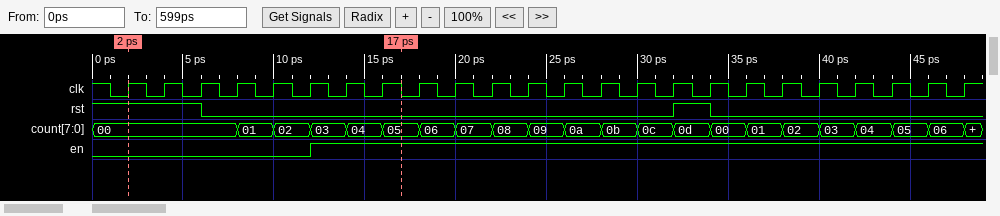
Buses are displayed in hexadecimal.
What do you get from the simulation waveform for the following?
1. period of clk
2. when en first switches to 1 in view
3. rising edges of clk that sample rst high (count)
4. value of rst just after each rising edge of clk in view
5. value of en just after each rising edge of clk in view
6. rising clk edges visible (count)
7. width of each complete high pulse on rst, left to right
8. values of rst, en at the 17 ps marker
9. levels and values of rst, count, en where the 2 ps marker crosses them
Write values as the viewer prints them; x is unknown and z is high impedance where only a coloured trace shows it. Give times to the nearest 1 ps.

2 ps
12 ps
4
1 1 0 0 0 0 0 0 0 0 0 0 0 0 0 1 0 0 0 0 0 0 0 0
0 0 0 0 0 1 1 1 1 1 1 1 1 1 1 1 1 1 1 1 1 1 1 1
24
2 ps
rst=0, en=1
rst=1, count=00, en=0
